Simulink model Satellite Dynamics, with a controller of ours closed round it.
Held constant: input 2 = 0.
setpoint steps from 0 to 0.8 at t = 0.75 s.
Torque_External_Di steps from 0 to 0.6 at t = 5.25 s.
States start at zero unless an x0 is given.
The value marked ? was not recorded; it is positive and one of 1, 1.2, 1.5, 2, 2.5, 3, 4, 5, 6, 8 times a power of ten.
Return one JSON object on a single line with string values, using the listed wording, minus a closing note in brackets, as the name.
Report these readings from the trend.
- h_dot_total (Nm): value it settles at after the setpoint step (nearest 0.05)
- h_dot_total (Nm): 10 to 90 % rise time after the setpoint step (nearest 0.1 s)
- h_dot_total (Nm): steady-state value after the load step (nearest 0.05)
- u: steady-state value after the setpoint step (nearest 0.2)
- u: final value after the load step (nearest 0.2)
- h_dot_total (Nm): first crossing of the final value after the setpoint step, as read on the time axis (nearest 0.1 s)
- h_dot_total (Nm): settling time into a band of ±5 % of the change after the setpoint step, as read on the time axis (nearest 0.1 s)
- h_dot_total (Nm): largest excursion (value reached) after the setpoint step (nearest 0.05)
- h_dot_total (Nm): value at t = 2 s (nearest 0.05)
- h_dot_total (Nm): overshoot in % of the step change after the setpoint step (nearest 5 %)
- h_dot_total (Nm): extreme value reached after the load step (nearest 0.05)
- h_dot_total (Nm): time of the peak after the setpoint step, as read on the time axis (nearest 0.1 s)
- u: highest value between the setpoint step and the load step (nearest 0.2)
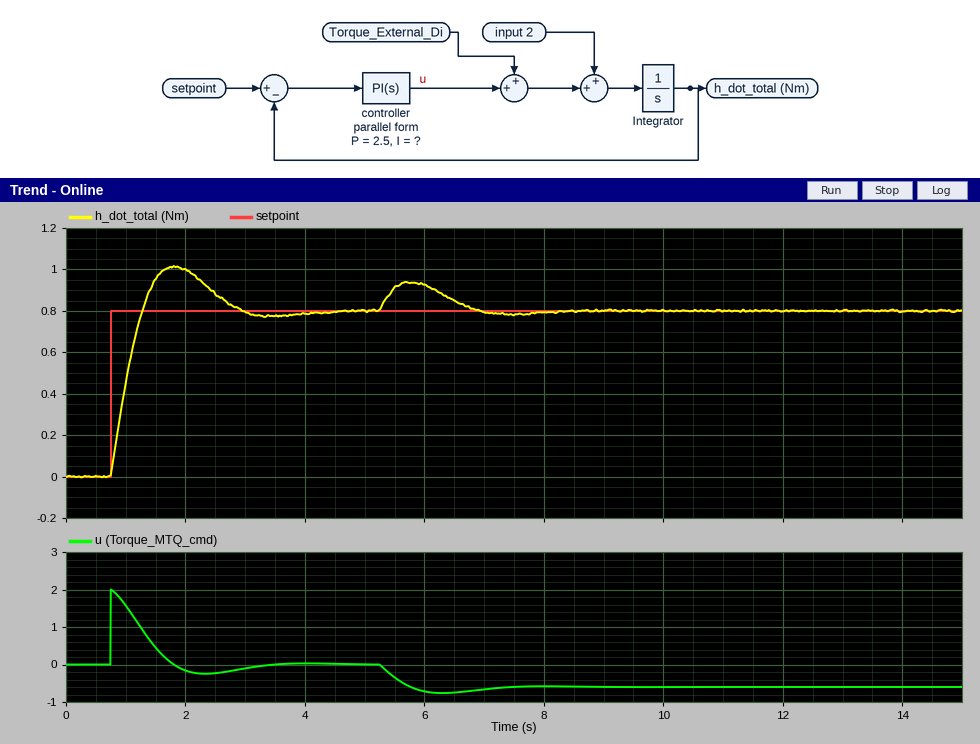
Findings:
{"h_dot_total (Nm): value it settles at after the setpoint step": "0.80", "h_dot_total (Nm): 10 to 90 % rise time after the setpoint step": "0.4 s", "h_dot_total (Nm): steady-state value after the load step": "0.80", "u: steady-state value after the setpoint step": "0.0", "u: final value after the load step": "-0.6", "h_dot_total (Nm): first crossing of the final value after the setpoint step, as read on the time axis": "1.3 s", "h_dot_total (Nm): settling time into a band of ±5 % of the change after the setpoint step, as read on the time axis": "2.7 s", "h_dot_total (Nm): largest excursion (value reached) after the setpoint step": "1.00", "h_dot_total (Nm): value at t = 2 s": "1.00", "h_dot_total (Nm): overshoot in % of the step change after the setpoint step": "25 %", "h_dot_total (Nm): extreme value reached after the load step": "0.95", "h_dot_total (Nm): time of the peak after the setpoint step, as read on the time axis": "1.8 s", "u: highest value between the setpoint step and the load step": "2.0"}
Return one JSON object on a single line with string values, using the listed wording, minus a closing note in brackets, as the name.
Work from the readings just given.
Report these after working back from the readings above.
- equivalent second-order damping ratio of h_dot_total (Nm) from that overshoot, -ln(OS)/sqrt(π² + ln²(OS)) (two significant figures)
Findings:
{"equivalent second-order damping ratio of h_dot_total (Nm) from that overshoot, -ln(OS)/sqrt(π² + ln²(OS))": "0.40"}
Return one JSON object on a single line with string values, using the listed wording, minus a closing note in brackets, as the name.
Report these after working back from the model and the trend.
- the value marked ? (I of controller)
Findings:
{"the value marked ?": "5"}
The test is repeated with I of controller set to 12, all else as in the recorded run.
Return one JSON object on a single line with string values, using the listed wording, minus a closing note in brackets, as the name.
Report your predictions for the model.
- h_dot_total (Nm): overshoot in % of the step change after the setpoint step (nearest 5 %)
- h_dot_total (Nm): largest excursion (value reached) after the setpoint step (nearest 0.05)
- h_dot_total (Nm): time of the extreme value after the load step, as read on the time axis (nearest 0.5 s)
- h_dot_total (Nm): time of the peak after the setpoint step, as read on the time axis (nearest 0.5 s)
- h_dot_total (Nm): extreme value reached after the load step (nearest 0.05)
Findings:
{"h_dot_total (Nm): overshoot in % of the step change after the setpoint step": "40 %", "h_dot_total (Nm): largest excursion (value reached) after the setpoint step": "1.10", "h_dot_total (Nm): time of the extreme value after the load step, as read on the time axis": "5.5 s", "h_dot_total (Nm): time of the peak after the setpoint step, as read on the time axis": "1.5 s", "h_dot_total (Nm): extreme value reached after the load step": "0.90"}
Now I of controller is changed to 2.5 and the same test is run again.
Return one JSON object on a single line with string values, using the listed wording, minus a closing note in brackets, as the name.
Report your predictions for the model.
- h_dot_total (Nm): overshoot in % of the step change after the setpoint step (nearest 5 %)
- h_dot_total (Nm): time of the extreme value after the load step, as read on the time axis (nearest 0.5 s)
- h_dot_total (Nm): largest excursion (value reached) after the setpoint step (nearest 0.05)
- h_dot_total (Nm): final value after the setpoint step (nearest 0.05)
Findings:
{"h_dot_total (Nm): overshoot in % of the step change after the setpoint step": "20 %", "h_dot_total (Nm): time of the extreme value after the load step, as read on the time axis": "6.0 s", "h_dot_total (Nm): largest excursion (value reached) after the setpoint step": "0.95", "h_dot_total (Nm): final value after the setpoint step": "0.80"}
